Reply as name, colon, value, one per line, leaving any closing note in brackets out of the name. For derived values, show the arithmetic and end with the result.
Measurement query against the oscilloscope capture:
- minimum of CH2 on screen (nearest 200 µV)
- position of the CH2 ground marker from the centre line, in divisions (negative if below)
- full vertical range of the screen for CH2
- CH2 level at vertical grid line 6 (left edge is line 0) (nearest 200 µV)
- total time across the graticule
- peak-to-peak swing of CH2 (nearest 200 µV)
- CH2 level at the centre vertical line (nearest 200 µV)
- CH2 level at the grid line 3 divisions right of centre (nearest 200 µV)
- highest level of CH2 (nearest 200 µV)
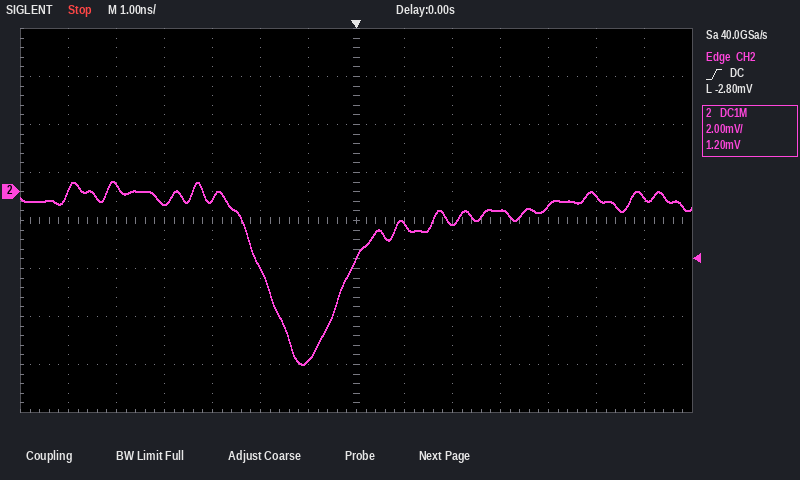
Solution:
minimum of CH2 on screen: -7.2 mV
position of the CH2 ground marker from the centre line, in divisions: +0.6 div
full vertical range of the screen for CH2: 16 mV
CH2 level at vertical grid line 6 (left edge is line 0): -7.0 mV
total time across the graticule: 14 ns
peak-to-peak swing of CH2: 400 µV − (-7.2 mV) = 7.6 mV
CH2 level at the centre vertical line: -2.8 mV
CH2 level at the grid line 3 divisions right of centre: -800 µV
highest level of CH2: 400 µV
